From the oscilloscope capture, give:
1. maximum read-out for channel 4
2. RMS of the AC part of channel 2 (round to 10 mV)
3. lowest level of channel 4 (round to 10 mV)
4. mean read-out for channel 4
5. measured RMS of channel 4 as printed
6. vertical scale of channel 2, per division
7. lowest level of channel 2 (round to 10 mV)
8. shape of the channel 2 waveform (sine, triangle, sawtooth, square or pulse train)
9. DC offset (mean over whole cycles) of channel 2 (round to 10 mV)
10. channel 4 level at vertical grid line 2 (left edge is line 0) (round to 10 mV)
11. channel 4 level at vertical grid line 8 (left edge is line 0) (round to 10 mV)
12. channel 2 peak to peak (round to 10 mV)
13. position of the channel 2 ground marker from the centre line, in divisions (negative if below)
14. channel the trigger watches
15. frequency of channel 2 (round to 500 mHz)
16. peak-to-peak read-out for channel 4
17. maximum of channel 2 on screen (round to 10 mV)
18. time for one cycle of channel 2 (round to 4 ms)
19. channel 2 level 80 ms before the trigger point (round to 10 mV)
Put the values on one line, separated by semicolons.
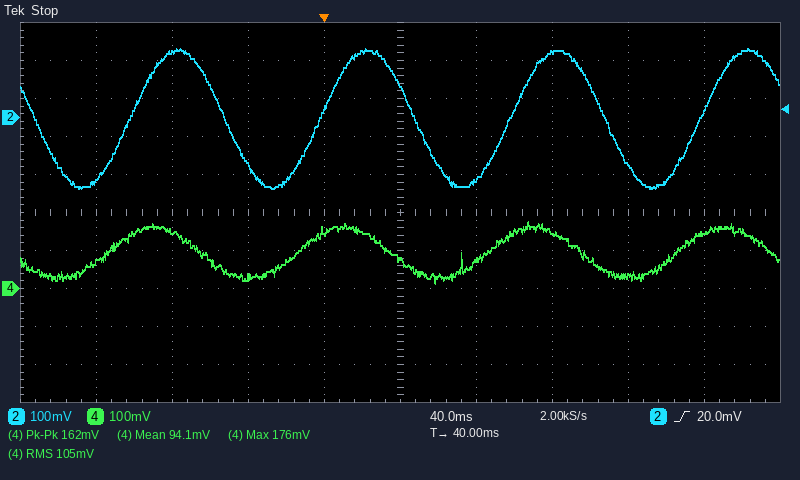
176 mV; 130 mV; 10 mV; 94.1 mV; 105 mV; 100 mV; -190 mV; sine; 0 mV; 150 mV; 30 mV; 370 mV; +2.5 div; channel 2; 10.0 Hz; 162 mV; 180 mV; 100 ms; 170 mV
